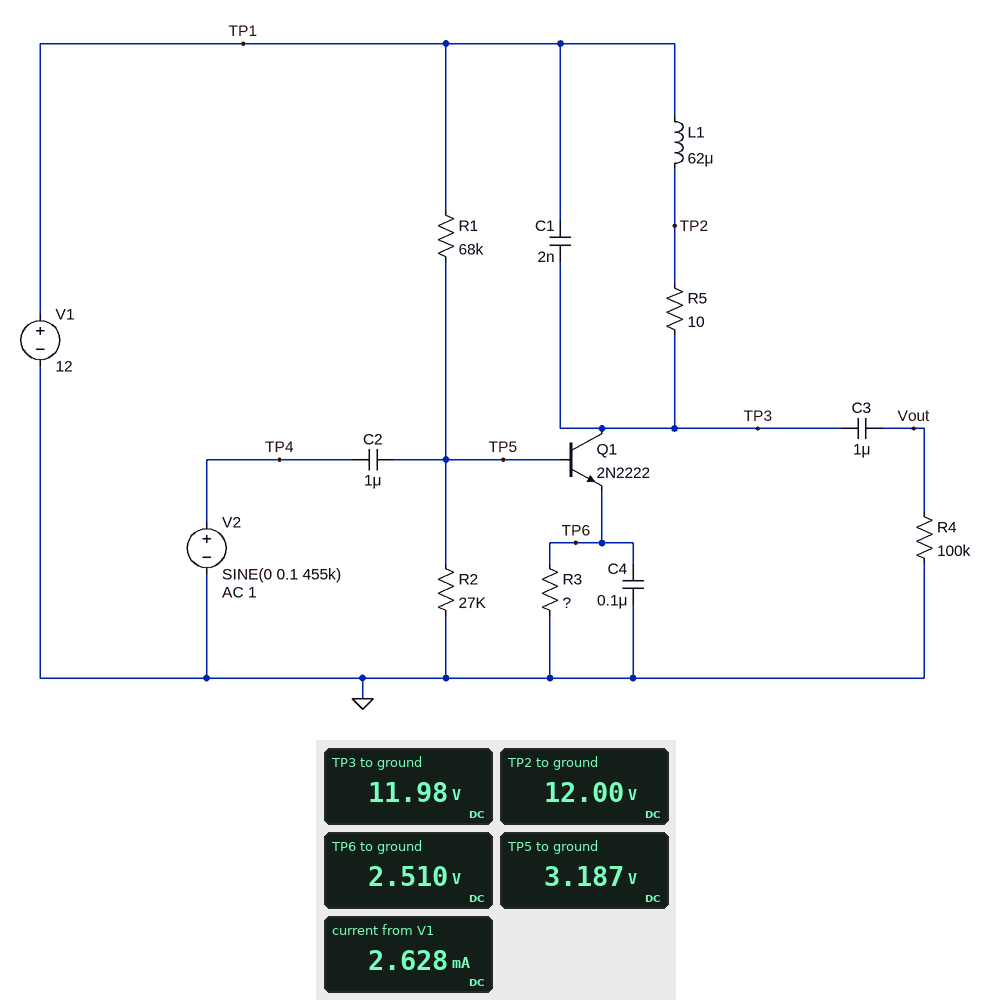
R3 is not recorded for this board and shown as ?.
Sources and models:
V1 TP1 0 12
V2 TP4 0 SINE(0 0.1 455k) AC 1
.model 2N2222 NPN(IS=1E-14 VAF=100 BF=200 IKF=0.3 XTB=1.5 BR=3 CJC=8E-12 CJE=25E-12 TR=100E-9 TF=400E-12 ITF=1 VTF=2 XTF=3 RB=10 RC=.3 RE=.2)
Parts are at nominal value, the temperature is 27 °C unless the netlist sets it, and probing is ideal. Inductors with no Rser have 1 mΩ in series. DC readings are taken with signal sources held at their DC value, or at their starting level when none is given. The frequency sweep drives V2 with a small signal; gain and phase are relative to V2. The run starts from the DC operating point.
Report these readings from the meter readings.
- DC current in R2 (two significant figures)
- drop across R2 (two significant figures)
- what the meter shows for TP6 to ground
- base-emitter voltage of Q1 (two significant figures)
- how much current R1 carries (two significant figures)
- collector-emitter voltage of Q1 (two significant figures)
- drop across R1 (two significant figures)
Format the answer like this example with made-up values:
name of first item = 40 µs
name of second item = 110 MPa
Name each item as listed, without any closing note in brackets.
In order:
DC current in R2 = 120 µA
drop across R2 = 3.2 V
what the meter shows for TP6 to ground = 2.510 V
base-emitter voltage of Q1 = 680 mV
how much current R1 carries = 130 µA
collector-emitter voltage of Q1 = 9.5 V
drop across R1 = 8.8 V
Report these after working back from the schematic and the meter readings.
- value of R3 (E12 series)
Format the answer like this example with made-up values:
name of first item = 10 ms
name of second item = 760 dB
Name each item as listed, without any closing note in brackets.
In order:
value of R3 = 1 kΩ
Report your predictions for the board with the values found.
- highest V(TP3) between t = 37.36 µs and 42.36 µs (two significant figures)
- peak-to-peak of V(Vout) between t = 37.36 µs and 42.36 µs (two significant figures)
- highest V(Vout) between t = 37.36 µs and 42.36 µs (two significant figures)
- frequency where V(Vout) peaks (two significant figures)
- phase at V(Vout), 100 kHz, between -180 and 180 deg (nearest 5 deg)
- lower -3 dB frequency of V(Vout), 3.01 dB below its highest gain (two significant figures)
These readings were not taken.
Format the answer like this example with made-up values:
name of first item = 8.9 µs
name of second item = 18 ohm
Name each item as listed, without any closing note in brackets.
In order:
highest V(TP3) between t = 37.36 µs and 42.36 µs = 22 V
peak-to-peak of V(Vout) between t = 37.36 µs and 42.36 µs = 19 V
highest V(Vout) between t = 37.36 µs and 42.36 µs = 9.9 V
frequency where V(Vout) peaks = 450 kHz
phase at V(Vout), 100 kHz, between -180 and 180 deg = -50 deg
lower -3 dB frequency of V(Vout), 3.01 dB below its highest gain = 440 kHz
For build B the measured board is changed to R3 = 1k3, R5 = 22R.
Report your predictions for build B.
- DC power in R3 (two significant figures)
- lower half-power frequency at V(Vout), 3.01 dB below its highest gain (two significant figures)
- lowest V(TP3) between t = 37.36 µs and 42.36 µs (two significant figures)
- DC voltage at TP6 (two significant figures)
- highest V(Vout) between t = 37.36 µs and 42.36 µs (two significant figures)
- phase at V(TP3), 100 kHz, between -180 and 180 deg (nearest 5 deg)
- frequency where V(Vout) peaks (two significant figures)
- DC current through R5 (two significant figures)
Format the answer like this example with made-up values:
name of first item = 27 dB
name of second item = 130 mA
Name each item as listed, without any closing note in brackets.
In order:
DC power in R3 = 5.1 mW
lower half-power frequency at V(Vout), 3.01 dB below its highest gain = 420 kHz
lowest V(TP3) between t = 37.36 µs and 42.36 µs = 7.0 V
DC voltage at TP6 = 2.6 V
highest V(Vout) between t = 37.36 µs and 42.36 µs = 4.6 V
phase at V(TP3), 100 kHz, between -180 and 180 deg = -70 deg
frequency where V(Vout) peaks = 450 kHz
DC current through R5 = 2.0 mA
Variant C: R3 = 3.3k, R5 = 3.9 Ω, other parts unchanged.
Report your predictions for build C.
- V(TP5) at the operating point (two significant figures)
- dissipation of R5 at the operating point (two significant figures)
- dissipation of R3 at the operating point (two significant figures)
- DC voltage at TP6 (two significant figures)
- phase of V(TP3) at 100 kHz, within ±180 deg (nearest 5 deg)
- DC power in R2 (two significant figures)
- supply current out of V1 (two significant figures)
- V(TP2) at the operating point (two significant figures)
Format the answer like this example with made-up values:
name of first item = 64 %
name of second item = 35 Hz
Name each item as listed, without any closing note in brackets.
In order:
V(TP5) at the operating point = 3.3 V
dissipation of R5 at the operating point = 2.6 µW
dissipation of R3 at the operating point = 2.2 mW
DC voltage at TP6 = 2.7 V
phase of V(TP3) at 100 kHz, within ±180 deg = -70 deg
DC power in R2 = 410 µW
supply current out of V1 = 940 µA
V(TP2) at the operating point = 12 V
